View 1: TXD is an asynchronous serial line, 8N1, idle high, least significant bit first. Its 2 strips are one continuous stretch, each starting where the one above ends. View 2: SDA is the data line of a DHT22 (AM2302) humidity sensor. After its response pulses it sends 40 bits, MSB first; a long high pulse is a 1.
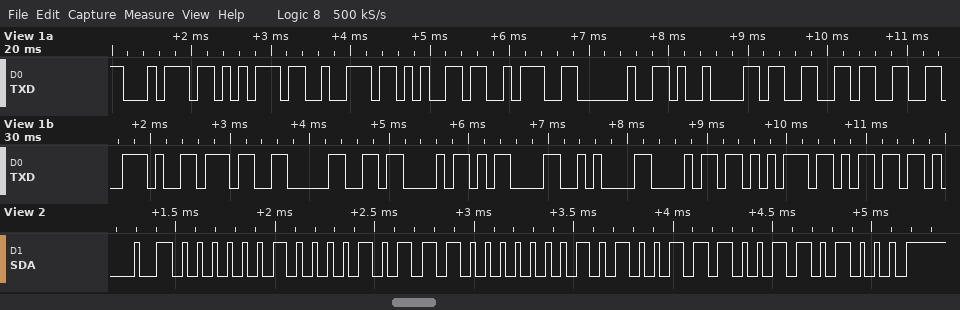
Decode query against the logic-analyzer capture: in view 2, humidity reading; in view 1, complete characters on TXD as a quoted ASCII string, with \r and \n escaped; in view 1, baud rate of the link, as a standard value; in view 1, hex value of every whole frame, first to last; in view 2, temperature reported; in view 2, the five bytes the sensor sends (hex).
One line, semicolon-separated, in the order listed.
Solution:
53.5 %; "ture: \t33.70C\r\nhum"; 9600 baud; 0x74 0x75 0x72 0x65 0x3A 0x20 0x09 0x33 0x33 0x2E 0x37 0x30 0x43 0x0D 0x0A 0x68 0x75 0x6D; 33.4 °C; 02 17 01 4E 68
